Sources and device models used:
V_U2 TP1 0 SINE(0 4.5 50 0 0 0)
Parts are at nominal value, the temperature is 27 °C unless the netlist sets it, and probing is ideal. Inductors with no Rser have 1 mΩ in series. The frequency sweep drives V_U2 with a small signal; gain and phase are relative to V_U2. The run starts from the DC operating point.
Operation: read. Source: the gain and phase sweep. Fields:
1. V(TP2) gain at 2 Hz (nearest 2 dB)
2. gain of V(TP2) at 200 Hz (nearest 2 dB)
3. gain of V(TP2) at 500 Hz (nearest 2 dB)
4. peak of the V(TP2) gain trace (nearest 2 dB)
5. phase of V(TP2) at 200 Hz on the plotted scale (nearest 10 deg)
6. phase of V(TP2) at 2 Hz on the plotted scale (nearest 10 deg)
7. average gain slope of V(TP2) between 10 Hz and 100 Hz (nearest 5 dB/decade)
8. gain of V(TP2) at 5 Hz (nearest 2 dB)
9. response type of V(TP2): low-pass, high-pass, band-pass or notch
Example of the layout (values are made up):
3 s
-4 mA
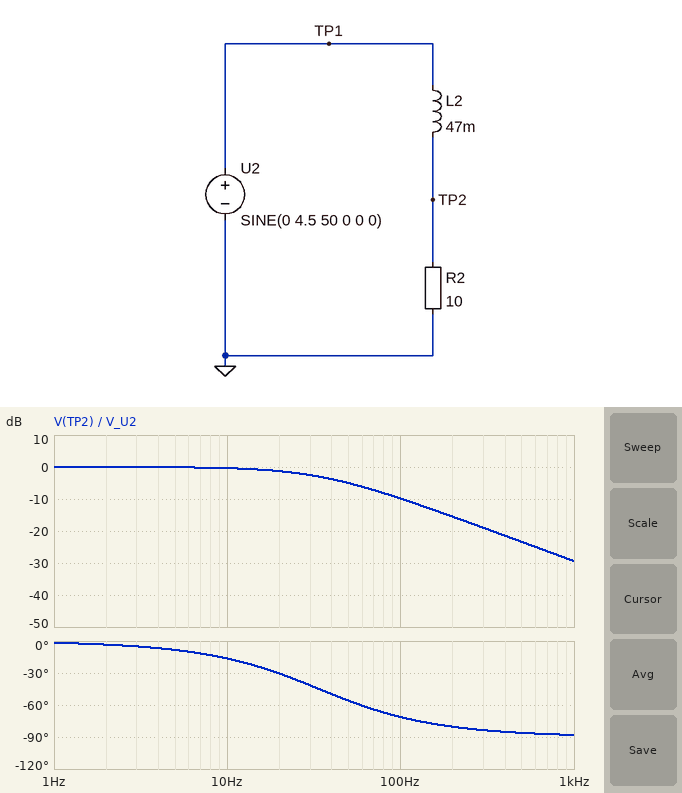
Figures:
0 dB
-16 dB
-24 dB
0 dB
-80 deg
0 deg
-10 dB/decade
0 dB
low-pass
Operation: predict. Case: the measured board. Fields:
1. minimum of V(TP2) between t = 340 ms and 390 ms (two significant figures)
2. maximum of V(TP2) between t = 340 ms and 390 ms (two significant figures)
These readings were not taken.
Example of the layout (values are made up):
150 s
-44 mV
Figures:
-2.5 V
2.5 V
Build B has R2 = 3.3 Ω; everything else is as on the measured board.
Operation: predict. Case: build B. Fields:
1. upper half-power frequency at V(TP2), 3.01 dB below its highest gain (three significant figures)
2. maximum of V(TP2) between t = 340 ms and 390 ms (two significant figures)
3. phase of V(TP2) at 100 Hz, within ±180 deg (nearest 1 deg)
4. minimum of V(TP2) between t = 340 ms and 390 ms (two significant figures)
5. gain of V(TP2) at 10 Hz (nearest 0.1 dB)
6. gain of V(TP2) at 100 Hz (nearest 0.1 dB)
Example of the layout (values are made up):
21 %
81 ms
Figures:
11.2 Hz
980 mV
-84 deg
-980 mV
-2.6 dB
-19.1 dB
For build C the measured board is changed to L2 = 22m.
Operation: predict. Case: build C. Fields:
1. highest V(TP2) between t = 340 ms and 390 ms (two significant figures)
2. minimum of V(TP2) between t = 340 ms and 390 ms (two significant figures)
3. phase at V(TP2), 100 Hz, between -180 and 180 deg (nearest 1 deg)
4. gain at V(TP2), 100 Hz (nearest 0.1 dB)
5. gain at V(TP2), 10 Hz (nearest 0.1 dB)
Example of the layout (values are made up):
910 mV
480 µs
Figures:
3.7 V
-3.7 V
-54 deg
-4.6 dB
-0.1 dB
